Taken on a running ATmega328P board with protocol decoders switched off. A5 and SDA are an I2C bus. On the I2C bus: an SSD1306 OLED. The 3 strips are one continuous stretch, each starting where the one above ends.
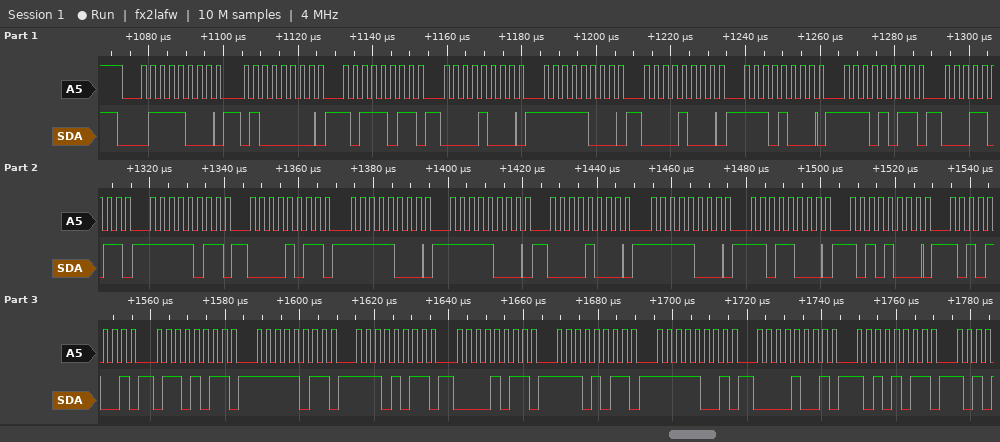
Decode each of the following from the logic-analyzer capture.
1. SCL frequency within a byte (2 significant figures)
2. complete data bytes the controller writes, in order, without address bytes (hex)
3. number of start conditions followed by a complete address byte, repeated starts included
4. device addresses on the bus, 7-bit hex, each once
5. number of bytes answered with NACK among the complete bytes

400 kHz
40 BB 08 F8 08 E8 EB 1B FB 0B F8 F8 08 F8 D8 A8 A9 6B FB EB 0B EB F9 09 AB
1
0x3C
0
